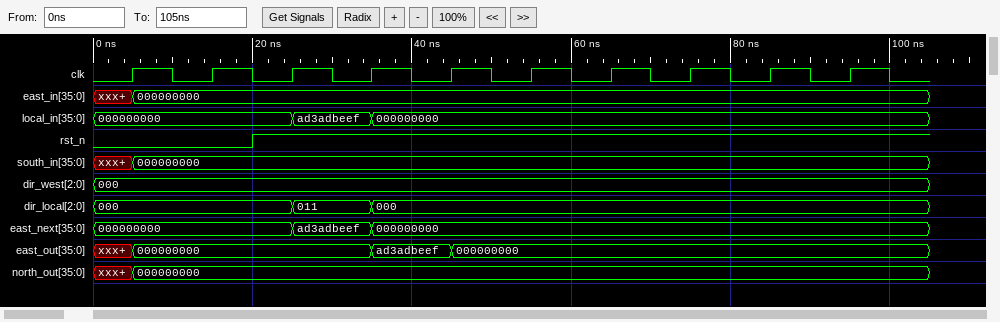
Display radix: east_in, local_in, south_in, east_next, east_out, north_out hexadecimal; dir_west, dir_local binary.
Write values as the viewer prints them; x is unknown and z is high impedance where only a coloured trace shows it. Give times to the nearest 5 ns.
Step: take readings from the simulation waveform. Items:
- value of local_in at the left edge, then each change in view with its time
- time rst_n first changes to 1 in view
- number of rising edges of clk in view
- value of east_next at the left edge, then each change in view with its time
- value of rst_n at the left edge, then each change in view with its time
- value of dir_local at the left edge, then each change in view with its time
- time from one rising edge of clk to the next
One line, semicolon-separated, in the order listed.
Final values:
000000000, ad3adbeef at 25 ns, 000000000 at 35 ns; 20 ns; 10; 000000000, ad3adbeef at 25 ns, 000000000 at 35 ns; 0, 1 at 20 ns; 000, 011 at 25 ns, 000 at 35 ns; 10 ns
